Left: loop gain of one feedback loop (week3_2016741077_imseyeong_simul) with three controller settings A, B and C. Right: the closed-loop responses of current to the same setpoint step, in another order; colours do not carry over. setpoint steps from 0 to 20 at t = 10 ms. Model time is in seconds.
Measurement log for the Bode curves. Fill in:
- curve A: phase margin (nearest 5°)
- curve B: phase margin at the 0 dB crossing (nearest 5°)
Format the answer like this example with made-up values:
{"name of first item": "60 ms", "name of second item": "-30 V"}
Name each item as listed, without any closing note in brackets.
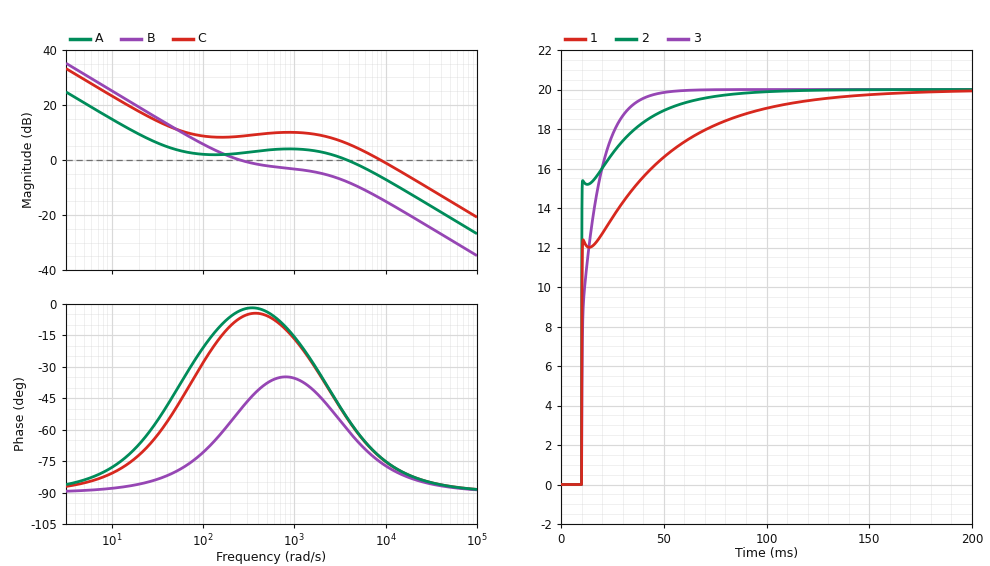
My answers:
{"curve A: phase margin": "125°", "curve B: phase margin at the 0 dB crossing": "130°"}
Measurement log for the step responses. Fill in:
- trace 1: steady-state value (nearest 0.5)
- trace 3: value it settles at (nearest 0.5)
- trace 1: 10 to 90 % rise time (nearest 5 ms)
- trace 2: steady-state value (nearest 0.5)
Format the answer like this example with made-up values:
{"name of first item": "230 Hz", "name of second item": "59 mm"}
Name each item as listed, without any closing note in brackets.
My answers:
{"trace 1: steady-state value": "20.0", "trace 3: value it settles at": "20.0", "trace 1: 10 to 90 % rise time": "60 ms", "trace 2: steady-state value": "20.0"}
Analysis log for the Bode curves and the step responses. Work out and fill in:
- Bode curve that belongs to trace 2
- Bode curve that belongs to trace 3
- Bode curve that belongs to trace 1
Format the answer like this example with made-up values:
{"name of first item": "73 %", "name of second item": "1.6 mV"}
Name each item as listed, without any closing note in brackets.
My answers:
{"Bode curve that belongs to trace 2": "C", "Bode curve that belongs to trace 3": "B", "Bode curve that belongs to trace 1": "A"}
